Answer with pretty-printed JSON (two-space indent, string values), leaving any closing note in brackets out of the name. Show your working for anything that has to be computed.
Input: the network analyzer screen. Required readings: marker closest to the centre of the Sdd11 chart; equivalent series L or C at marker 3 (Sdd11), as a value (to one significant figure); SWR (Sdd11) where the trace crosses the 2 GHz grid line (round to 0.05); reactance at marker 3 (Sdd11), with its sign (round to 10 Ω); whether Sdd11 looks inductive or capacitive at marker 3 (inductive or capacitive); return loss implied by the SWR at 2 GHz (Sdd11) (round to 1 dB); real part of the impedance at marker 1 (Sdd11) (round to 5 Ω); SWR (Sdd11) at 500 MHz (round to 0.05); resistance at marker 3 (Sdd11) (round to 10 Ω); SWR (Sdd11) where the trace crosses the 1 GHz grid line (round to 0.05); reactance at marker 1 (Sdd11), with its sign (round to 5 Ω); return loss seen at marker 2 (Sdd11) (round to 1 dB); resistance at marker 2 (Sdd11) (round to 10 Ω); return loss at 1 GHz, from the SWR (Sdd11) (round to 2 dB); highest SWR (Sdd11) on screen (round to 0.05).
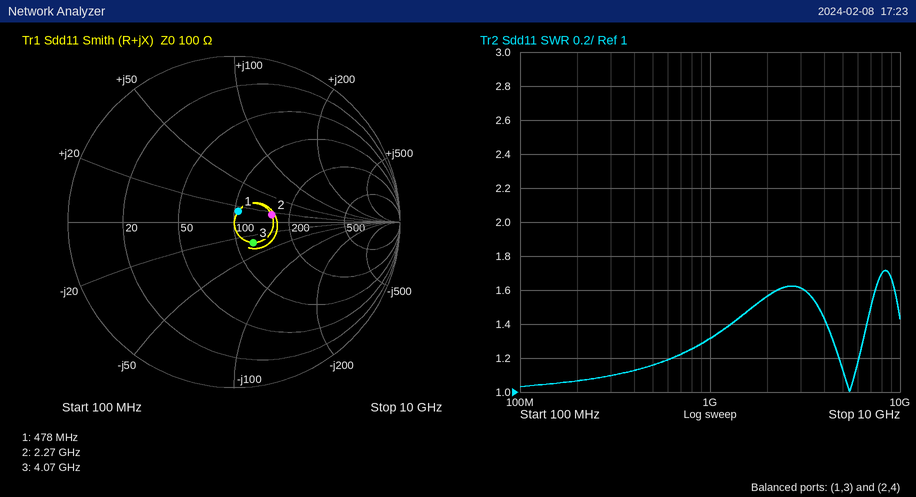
{
  "marker closest to the centre of the Sdd11 chart": "marker 1",
  "equivalent series L or C at marker 3 (Sdd11), as a value": "C = 1/(2π × 4.07 GHz × 30 Ω) ≈ 1 pF",
  "SWR (Sdd11) where the trace crosses the 2 GHz grid line": "1.55",
  "reactance at marker 3 (Sdd11), with its sign": "-30 Ω",
  "whether Sdd11 looks inductive or capacitive at marker 3": "capacitive",
  "return loss implied by the SWR at 2 GHz (Sdd11)": "−20 log10((1.55 − 1)/(1.55 + 1)) ≈ 13 dB",
  "real part of the impedance at marker 1 (Sdd11)": "105 Ω",
  "SWR (Sdd11) at 500 MHz": "1.15",
  "resistance at marker 3 (Sdd11)": "120 Ω",
  "SWR (Sdd11) where the trace crosses the 1 GHz grid line": "1.30",
  "reactance at marker 1 (Sdd11), with its sign": "+15 Ω",
  "return loss seen at marker 2 (Sdd11)": "13 dB",
  "resistance at marker 2 (Sdd11)": "160 Ω",
  "return loss at 1 GHz, from the SWR (Sdd11)": "−20 log10((1.3 − 1)/(1.3 + 1)) ≈ 18 dB",
  "highest SWR (Sdd11) on screen": "1.70"
}
